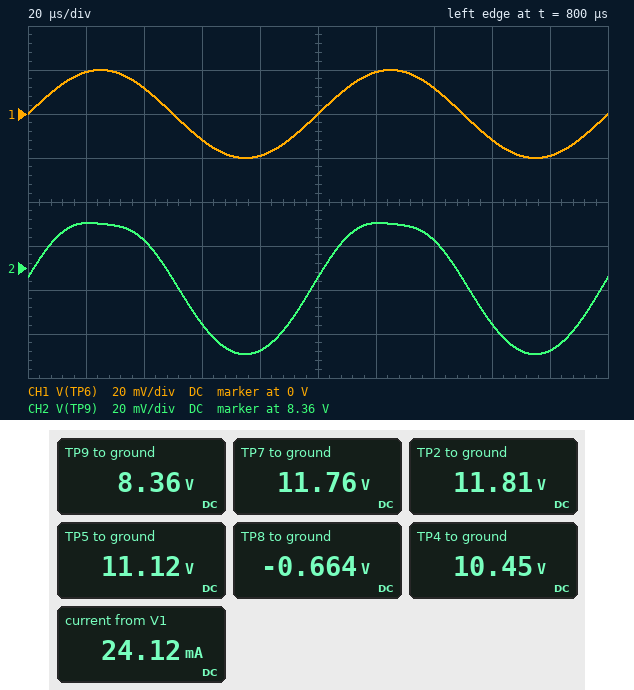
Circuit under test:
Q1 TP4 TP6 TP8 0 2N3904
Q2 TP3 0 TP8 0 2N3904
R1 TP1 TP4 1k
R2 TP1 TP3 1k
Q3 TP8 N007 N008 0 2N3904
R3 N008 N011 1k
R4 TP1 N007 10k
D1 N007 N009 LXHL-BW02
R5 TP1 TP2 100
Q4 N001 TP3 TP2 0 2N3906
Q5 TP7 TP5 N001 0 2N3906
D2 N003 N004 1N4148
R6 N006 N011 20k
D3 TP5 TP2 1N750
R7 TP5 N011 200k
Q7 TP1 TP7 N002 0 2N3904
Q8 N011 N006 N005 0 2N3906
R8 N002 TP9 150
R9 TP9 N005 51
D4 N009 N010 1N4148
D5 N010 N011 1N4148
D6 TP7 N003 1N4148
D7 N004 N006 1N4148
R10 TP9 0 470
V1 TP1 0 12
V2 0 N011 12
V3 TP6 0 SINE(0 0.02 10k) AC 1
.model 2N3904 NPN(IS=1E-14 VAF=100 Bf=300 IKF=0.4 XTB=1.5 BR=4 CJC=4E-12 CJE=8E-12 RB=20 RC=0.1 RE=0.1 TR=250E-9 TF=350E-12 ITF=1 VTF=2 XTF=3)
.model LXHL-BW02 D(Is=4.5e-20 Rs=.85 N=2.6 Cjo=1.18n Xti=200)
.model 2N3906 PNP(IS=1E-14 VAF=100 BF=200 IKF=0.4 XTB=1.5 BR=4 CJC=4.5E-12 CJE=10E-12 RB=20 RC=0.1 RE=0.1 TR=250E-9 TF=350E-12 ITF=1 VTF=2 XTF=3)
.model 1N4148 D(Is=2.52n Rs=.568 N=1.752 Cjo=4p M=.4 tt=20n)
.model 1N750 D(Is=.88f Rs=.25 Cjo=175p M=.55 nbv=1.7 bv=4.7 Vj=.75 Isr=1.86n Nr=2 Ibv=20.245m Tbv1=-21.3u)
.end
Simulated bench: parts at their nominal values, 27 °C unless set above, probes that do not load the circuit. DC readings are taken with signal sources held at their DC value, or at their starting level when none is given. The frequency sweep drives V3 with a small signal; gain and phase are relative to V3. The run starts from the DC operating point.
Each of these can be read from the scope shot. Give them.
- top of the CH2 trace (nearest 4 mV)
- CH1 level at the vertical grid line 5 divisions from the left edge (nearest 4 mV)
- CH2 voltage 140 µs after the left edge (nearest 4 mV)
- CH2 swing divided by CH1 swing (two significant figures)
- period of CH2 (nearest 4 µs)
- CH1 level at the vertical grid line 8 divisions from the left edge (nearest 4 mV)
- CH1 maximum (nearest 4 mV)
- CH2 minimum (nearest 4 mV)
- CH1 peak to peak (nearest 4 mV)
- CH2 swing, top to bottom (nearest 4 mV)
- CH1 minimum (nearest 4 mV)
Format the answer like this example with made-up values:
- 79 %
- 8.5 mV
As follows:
- 8.380 V
- 0 V
- 8.372 V
- 1.5
- 100 µs
- -12 mV
- 20 mV
- 8.320 V
- 40 mV
- 60 mV
- -20 mV
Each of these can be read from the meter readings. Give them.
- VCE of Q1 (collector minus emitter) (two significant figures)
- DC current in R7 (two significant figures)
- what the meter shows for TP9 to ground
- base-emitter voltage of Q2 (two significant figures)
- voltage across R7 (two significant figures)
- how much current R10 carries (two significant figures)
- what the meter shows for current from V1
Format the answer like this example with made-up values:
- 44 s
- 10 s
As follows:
- 11 V
- 120 µA
- 8.36 V
- 660 mV
- 23 V
- 18 mA
- 24.12 mA
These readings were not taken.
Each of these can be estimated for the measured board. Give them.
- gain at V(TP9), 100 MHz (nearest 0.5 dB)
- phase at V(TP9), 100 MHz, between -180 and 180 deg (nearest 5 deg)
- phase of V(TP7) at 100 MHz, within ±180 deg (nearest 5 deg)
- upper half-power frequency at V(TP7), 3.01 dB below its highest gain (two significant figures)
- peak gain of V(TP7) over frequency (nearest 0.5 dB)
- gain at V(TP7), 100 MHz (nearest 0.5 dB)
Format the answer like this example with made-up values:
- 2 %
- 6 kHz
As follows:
- 1.0 dB
- -55 deg
- -55 deg
- 56 MHz
- 9.0 dB
- 3.0 dB
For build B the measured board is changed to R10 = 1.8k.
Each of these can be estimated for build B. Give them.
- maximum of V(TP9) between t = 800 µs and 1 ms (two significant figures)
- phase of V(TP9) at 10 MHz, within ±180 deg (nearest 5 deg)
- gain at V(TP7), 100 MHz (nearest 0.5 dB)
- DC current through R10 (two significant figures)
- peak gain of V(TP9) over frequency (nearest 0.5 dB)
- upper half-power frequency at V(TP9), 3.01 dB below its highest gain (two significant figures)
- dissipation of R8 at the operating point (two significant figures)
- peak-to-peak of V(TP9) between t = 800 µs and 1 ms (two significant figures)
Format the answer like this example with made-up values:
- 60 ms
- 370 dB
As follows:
- 10 V
- -10 deg
- 3.5 dB
- 5.7 mA
- 8.0 dB
- 61 MHz
- 4.8 mW
- 73 mV
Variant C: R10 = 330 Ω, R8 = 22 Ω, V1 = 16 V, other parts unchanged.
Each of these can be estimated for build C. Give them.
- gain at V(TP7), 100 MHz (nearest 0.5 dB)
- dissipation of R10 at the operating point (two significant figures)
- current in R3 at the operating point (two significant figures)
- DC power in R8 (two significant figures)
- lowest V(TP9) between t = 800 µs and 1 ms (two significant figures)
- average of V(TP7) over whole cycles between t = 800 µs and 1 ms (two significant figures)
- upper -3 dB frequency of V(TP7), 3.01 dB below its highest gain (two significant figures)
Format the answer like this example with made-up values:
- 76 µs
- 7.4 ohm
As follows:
- 3.5 dB
- 600 mW
- 3.2 mA
- 40 mW
- 14 V
- 16 V
- 62 MHz
